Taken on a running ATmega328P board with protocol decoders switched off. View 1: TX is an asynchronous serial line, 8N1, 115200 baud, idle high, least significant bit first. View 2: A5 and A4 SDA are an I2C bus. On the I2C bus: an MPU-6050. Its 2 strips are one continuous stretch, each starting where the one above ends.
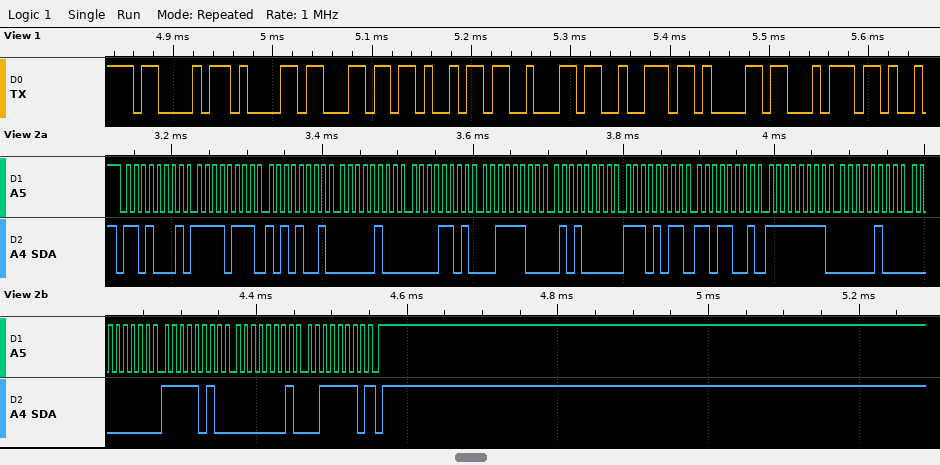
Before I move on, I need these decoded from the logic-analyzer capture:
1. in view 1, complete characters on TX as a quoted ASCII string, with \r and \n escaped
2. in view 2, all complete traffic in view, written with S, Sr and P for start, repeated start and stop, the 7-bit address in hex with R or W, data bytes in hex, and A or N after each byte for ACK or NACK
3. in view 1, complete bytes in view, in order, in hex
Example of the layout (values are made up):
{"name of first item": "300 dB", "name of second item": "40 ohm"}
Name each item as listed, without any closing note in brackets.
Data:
{"in view 1, complete characters on TX as a quoted ASCII string, with \\r and \\n escaped": "\"Calibrat\"", "in view 2, all complete traffic in view, written with S, Sr and P for start, repeated start and stop, the 7-bit address in hex with R or W, data bytes in hex, and A or N after each byte for ACK or NACK": "S 68R A F7 A A9 A 04 A 0D A 3C A 50 A EB A D9 A FF A 04 A 00 A FA A 01 A 3E N P", "in view 1, complete bytes in view, in order, in hex": "43 61 6C 69 62 72 61 74"}
